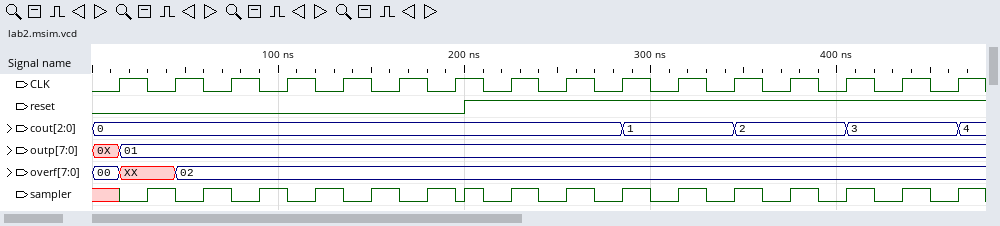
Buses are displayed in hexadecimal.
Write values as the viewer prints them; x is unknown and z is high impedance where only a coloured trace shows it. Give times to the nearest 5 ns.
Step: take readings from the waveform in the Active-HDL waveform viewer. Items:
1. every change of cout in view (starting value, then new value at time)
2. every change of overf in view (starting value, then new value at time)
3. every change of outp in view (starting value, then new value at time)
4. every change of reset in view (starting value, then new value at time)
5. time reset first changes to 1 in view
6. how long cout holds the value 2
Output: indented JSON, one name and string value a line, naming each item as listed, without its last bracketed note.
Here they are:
{
  "every change of cout in view": "0, 1 at 285 ns, 2 at 345 ns, 3 at 405 ns, 4 at 465 ns",
  "every change of overf in view": "00, XX at 15 ns, 02 at 45 ns",
  "every change of outp in view": "0X, 01 at 15 ns",
  "every change of reset in view": "0, 1 at 200 ns",
  "time reset first changes to 1 in view": "200 ns",
  "how long cout holds the value 2": "60 ns"
}
